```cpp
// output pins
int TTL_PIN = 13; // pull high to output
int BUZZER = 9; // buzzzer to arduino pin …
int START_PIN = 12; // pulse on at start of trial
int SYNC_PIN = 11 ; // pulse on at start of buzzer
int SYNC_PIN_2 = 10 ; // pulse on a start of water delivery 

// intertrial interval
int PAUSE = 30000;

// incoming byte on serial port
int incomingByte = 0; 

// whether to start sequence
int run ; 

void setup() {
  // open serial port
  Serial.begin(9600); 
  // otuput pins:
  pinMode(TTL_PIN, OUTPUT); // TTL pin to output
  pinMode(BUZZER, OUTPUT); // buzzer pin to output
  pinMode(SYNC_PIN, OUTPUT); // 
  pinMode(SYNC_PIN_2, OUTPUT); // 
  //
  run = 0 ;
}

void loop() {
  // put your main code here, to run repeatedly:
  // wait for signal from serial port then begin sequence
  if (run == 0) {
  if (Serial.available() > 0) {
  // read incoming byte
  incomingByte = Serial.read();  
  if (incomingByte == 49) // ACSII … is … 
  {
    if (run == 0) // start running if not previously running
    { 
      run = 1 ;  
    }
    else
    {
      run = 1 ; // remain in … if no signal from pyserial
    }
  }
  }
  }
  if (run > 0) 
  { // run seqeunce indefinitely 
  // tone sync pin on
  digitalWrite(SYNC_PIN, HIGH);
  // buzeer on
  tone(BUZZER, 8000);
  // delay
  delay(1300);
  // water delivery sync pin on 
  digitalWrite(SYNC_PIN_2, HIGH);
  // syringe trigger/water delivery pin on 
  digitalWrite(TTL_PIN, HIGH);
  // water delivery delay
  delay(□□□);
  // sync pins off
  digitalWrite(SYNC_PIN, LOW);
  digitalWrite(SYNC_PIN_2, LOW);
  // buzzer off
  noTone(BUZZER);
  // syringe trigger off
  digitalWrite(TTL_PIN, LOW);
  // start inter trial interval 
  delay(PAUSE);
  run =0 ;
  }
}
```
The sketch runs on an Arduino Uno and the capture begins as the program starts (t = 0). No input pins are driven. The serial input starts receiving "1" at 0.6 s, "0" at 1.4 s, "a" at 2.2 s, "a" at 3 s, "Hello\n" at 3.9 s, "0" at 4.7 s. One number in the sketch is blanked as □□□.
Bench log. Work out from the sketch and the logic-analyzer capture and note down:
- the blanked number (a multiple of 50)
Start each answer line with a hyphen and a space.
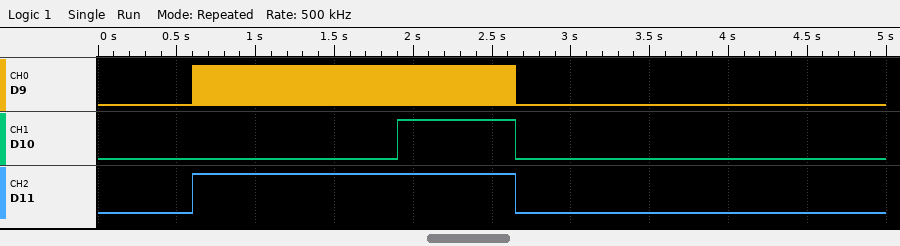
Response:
- 750
